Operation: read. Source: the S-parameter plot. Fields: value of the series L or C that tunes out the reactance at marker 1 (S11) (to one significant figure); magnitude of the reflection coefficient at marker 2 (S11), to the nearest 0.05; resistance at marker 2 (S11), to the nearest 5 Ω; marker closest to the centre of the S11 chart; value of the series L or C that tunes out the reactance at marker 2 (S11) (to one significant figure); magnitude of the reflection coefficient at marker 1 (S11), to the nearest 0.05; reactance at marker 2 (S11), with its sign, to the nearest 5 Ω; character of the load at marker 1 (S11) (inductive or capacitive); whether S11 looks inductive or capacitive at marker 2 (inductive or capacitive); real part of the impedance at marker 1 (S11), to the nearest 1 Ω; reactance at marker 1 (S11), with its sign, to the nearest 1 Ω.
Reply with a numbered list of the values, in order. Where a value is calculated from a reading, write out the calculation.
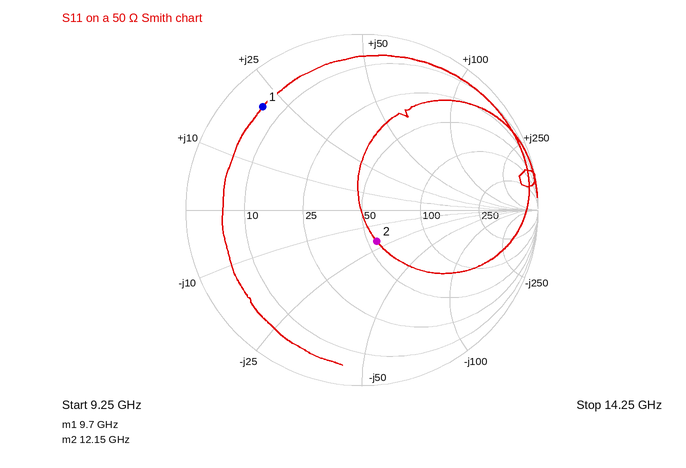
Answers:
1. C = 1/(2π × 9.7 GHz × 21 Ω) ≈ 781 fF, so 800 fF to one significant figure
2. 0.20
3. 55 Ω
4. marker 2
5. L = 20 Ω/(2π × 12.15 GHz) ≈ 262 pH, so 300 pH to one significant figure
6. 0.80
7. -20 Ω
8. inductive
9. capacitive
10. 6 Ω
11. +21 Ω
